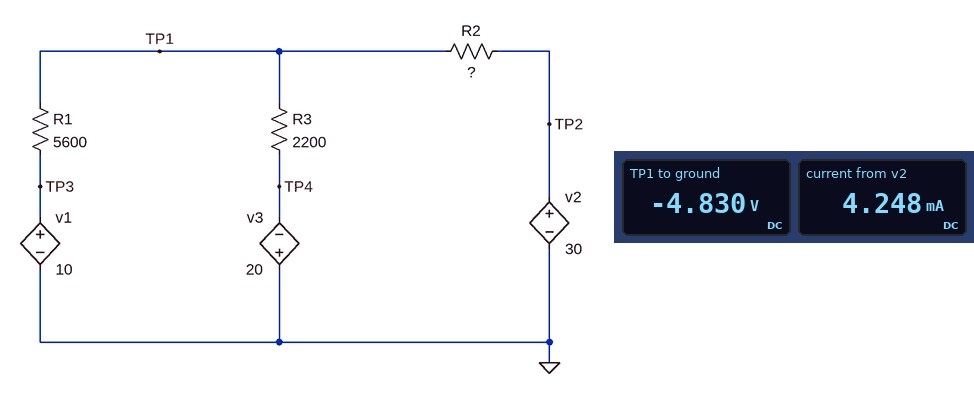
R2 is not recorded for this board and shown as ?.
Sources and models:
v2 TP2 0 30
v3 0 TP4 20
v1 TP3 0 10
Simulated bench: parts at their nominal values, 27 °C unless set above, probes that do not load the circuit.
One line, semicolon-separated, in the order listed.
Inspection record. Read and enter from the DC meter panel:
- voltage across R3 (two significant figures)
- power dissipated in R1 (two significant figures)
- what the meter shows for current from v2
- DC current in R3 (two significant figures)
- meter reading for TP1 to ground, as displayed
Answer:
15 V; 39 mW; 4.248 mA; 6.9 mA; -4.830 V
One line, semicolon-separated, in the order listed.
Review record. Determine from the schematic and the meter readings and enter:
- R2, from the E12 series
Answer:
8.2 kΩ
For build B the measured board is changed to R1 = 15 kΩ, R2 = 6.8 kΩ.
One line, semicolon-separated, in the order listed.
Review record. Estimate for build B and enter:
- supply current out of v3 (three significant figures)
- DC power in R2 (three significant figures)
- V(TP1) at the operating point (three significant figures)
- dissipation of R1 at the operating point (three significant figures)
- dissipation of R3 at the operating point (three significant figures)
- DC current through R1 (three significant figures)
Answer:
6.36 mA; 191 mW; -6.00 V; 17.1 mW; 89.0 mW; 1.07 mA
